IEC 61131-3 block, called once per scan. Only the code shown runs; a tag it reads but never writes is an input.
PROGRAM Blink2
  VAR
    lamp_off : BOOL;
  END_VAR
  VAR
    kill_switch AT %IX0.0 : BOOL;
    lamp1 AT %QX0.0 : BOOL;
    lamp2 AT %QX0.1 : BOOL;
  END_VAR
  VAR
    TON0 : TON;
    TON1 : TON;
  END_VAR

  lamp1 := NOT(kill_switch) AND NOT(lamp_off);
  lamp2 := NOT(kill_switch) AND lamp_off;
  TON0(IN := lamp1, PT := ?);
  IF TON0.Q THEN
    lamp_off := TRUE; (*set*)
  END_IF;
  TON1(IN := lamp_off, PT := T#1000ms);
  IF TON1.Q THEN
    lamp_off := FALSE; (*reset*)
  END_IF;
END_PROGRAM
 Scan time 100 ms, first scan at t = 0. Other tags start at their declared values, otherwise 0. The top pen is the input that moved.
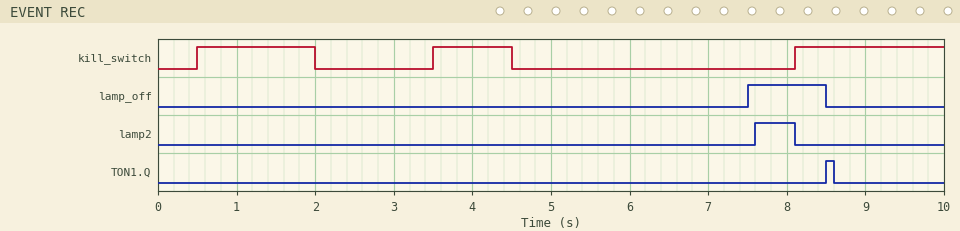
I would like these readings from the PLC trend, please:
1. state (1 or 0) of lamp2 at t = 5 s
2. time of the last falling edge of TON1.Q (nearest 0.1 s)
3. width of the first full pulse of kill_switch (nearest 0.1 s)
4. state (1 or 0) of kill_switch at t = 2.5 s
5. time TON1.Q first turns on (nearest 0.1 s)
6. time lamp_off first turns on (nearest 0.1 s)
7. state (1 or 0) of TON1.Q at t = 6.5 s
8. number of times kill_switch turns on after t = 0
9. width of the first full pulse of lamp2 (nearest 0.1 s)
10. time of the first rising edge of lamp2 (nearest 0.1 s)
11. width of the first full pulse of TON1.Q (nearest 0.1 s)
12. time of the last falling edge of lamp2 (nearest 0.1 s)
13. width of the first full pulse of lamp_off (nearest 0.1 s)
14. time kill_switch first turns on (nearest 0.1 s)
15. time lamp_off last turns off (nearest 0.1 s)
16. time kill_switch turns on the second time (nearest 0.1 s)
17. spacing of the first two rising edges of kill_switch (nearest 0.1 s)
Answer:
0
8.6 s
1.5 s
0
8.5 s
7.5 s
0
3
0.5 s
7.6 s
0.1 s
8.1 s
1.0 s
0.5 s
8.5 s
3.5 s
3.0 s
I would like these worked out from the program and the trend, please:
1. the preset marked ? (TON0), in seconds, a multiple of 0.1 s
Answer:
3.0 s
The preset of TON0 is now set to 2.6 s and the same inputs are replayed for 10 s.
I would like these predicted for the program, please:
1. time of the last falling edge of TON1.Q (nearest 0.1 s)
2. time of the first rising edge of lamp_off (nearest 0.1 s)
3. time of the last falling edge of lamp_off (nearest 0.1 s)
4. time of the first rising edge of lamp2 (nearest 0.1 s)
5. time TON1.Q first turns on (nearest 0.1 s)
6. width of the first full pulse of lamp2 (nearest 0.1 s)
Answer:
8.2 s
7.1 s
8.1 s
7.2 s
8.1 s
0.9 s
